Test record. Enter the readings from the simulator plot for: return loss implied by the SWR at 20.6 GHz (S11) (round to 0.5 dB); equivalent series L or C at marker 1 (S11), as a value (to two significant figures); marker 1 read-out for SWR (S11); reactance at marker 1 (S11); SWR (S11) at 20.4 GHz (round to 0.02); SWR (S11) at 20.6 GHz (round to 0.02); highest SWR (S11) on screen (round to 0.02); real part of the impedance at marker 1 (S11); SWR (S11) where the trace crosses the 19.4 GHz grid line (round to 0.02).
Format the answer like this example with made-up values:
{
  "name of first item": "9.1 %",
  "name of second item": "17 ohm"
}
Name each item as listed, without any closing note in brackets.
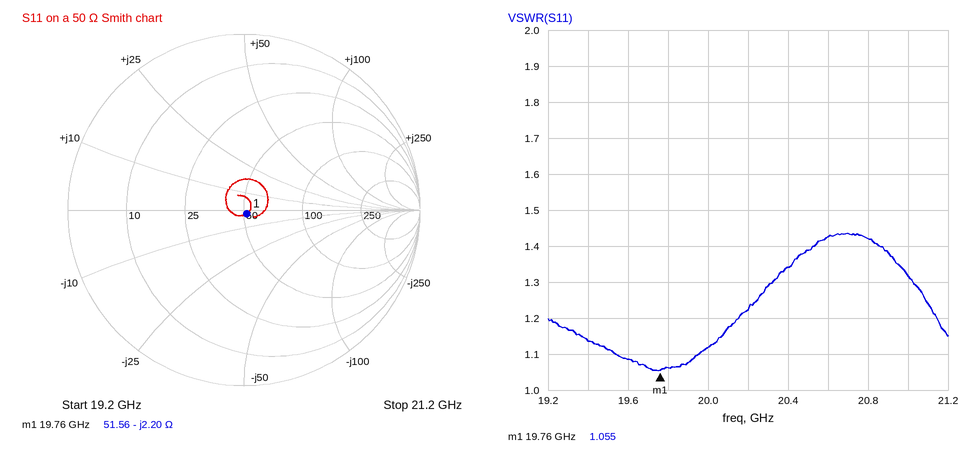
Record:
{
  "return loss implied by the SWR at 20.6 GHz (S11)": "15.0 dB",
  "equivalent series L or C at marker 1 (S11), as a value": "3.7 pF",
  "marker 1 read-out for SWR": "1.055",
  "reactance at marker 1": "-2.20 Ω",
  "SWR (S11) at 20.4 GHz": "1.34",
  "SWR (S11) at 20.6 GHz": "1.42",
  "highest SWR (S11) on screen": "1.44",
  "real part of the impedance at marker 1": "51.56 Ω",
  "SWR (S11) where the trace crosses the 19.4 GHz grid line": "1.14"
}
